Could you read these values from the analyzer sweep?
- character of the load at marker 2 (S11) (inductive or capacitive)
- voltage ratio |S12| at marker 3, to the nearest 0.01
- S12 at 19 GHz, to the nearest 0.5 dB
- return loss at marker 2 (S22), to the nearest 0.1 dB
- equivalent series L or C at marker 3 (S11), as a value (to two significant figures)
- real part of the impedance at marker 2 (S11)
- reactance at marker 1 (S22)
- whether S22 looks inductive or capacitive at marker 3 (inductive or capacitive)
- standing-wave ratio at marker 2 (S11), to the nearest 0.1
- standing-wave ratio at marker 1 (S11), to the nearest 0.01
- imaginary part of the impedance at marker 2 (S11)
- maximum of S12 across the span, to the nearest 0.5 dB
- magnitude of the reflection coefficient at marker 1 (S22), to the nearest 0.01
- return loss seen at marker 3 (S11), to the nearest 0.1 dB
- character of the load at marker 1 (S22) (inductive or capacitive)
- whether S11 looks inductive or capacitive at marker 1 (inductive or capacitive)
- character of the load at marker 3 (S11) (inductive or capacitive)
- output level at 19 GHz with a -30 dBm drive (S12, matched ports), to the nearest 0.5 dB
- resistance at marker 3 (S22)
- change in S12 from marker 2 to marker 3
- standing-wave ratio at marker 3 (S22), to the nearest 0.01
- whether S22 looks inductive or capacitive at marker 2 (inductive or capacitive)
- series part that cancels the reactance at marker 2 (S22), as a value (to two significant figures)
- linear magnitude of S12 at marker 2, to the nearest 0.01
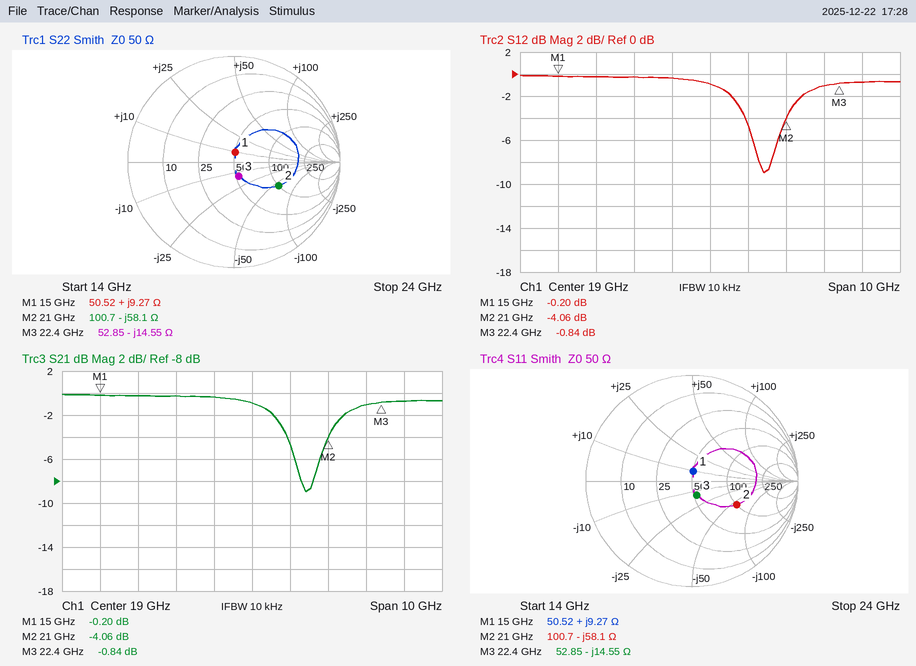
capacitive
0.91
-1.0 dB
6.4 dB
490 fF
100.7 Ω
+9.27 Ω
capacitive
2.8
1.20
-58.1 Ω
0.0 dB
0.09
16.9 dB
inductive
inductive
capacitive
-31.0 dBm
52.85 Ω
3.22 dB
1.33
capacitive
440 pH
0.63
